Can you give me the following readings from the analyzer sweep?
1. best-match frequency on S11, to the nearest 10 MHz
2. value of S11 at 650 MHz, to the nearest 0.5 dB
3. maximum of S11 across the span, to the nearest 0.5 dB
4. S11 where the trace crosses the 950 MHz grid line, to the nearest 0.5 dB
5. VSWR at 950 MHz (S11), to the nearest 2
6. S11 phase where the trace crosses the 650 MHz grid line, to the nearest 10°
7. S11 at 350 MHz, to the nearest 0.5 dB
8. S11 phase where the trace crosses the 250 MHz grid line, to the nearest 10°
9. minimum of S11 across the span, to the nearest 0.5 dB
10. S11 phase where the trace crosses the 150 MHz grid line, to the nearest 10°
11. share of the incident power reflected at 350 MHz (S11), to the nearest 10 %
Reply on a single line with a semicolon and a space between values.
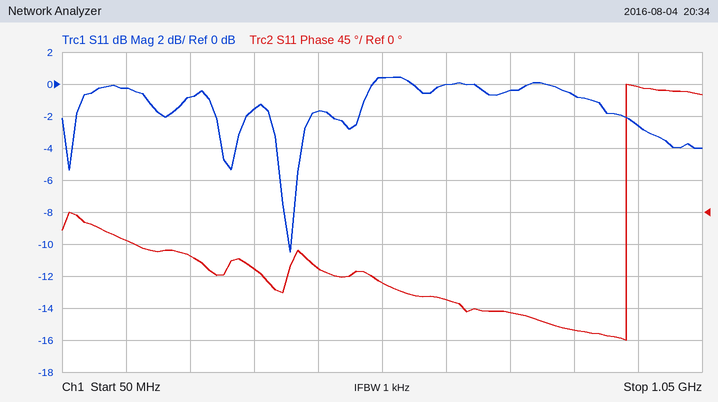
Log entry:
410 MHz; 0.0 dB; 0.5 dB; -2.5 dB; 6; -120°; -1.5 dB; -60°; -10.5 dB; -40°; 70 %
